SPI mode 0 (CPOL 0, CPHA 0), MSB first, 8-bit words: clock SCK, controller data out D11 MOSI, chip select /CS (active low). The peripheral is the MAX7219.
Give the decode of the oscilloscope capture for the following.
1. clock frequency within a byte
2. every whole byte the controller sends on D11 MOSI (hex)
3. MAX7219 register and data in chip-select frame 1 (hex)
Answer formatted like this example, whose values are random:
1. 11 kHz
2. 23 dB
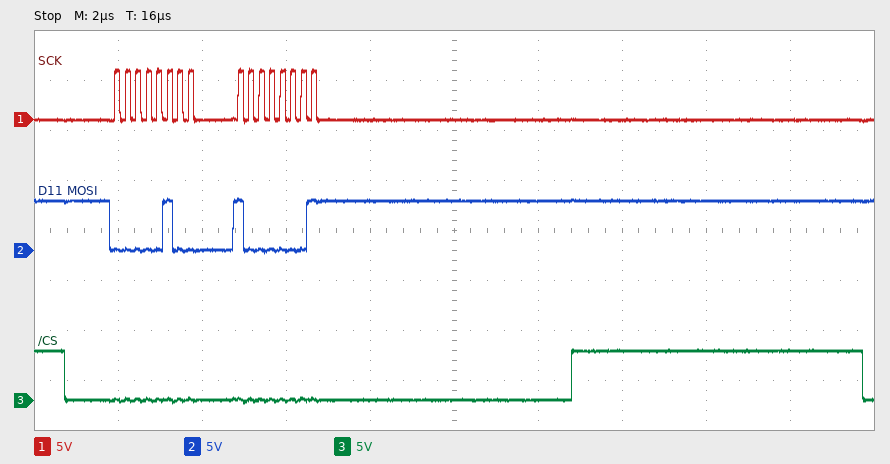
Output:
1. 4 MHz
2. 04 81
3. register 0x4, data 0x81
